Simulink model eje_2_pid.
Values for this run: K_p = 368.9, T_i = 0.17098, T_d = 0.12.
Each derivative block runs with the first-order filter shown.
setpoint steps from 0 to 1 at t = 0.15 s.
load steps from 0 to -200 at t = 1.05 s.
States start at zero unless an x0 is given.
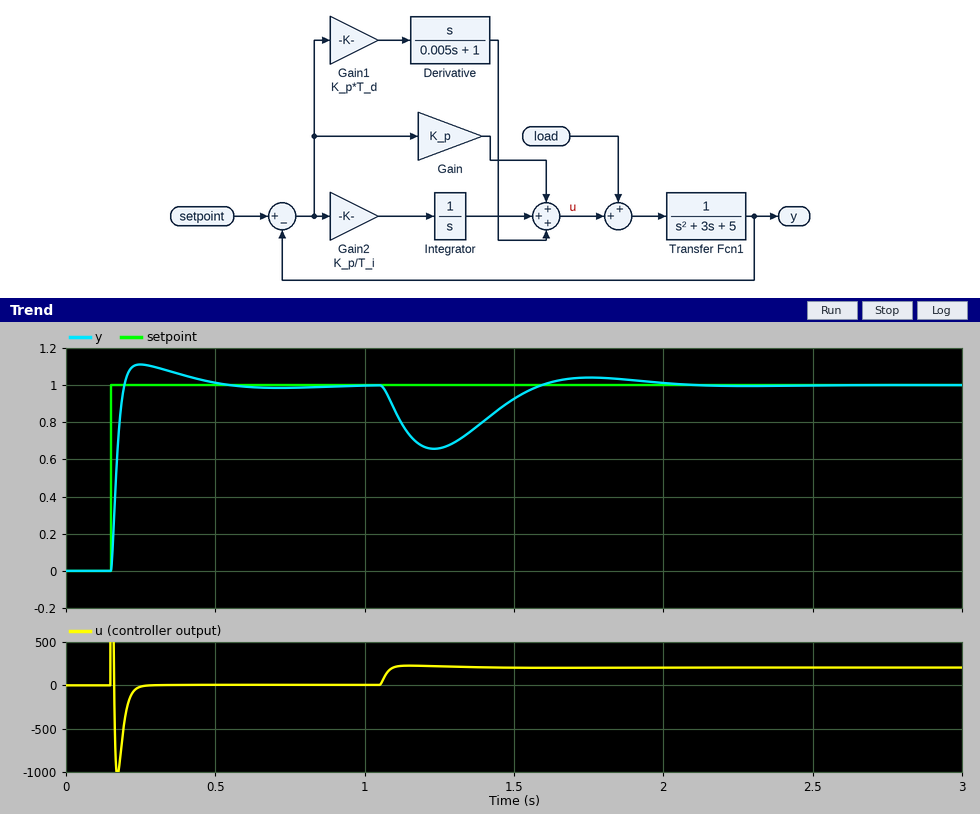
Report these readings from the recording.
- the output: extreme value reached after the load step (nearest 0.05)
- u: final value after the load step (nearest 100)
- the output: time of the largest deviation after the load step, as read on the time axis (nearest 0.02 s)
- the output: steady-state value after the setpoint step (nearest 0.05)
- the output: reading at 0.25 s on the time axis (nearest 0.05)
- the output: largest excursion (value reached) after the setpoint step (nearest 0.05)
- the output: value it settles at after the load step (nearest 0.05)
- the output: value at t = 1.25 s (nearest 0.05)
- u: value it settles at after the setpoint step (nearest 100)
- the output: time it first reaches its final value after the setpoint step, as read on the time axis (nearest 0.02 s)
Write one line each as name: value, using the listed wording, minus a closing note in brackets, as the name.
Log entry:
the output: extreme value reached after the load step: 0.65
u: final value after the load step: 200
the output: time of the largest deviation after the load step, as read on the time axis: 1.24 s
the output: steady-state value after the setpoint step: 1.00
the output: reading at 0.25 s on the time axis: 1.10
the output: largest excursion (value reached) after the setpoint step: 1.10
the output: value it settles at after the load step: 1.00
the output: value at t = 1.25 s: 0.65
u: value it settles at after the setpoint step: 0
the output: time it first reaches its final value after the setpoint step, as read on the time axis: 0.20 s
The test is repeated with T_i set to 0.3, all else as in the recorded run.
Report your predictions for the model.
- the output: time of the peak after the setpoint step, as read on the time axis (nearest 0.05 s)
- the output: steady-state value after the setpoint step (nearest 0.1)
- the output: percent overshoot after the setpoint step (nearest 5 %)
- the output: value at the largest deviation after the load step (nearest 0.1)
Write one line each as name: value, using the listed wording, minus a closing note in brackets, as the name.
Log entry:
the output: time of the peak after the setpoint step, as read on the time axis: 0.25 s
the output: steady-state value after the setpoint step: 1.0
the output: percent overshoot after the setpoint step: 10 %
the output: value at the largest deviation after the load step: 0.6
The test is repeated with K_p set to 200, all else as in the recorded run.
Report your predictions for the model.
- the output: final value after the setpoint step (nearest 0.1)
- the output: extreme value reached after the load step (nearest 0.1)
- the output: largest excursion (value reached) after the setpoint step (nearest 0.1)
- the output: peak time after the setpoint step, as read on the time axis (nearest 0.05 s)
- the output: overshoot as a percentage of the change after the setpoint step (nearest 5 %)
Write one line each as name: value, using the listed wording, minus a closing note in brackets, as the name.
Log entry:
the output: final value after the setpoint step: 1.0
the output: extreme value reached after the load step: 0.3
the output: largest excursion (value reached) after the setpoint step: 1.2
the output: peak time after the setpoint step, as read on the time axis: 0.30 s
the output: overshoot as a percentage of the change after the setpoint step: 20 %
